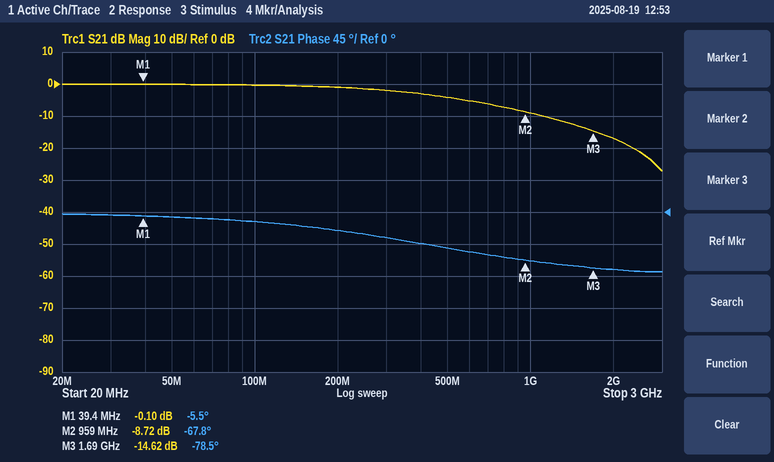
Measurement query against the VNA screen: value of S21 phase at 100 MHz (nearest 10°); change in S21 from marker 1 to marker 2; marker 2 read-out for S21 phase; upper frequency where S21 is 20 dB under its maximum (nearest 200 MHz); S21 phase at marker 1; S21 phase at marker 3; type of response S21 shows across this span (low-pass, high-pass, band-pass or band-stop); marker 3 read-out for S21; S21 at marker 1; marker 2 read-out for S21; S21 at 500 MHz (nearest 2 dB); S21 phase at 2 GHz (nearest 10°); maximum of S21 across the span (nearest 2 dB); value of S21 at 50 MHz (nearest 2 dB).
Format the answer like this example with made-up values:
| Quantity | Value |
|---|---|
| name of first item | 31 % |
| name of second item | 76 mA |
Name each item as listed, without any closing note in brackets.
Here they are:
| Quantity | Value |
|---|---|
| value of S21 phase at 100 MHz | -10° |
| change in S21 from marker 1 to marker 2 | -8.62 dB |
| marker 2 read-out for S21 phase | -67.8° |
| upper frequency where S21 is 20 dB under its maximum | 2.4 GHz |
| S21 phase at marker 1 | -5.5° |
| S21 phase at marker 3 | -78.5° |
| type of response S21 shows across this span | low-pass |
| marker 3 read-out for S21 | -14.62 dB |
| S21 at marker 1 | -0.10 dB |
| marker 2 read-out for S21 | -8.72 dB |
| S21 at 500 MHz | -4 dB |
| S21 phase at 2 GHz | -80° |
| maximum of S21 across the span | 0 dB |
| value of S21 at 50 MHz | 0 dB |
